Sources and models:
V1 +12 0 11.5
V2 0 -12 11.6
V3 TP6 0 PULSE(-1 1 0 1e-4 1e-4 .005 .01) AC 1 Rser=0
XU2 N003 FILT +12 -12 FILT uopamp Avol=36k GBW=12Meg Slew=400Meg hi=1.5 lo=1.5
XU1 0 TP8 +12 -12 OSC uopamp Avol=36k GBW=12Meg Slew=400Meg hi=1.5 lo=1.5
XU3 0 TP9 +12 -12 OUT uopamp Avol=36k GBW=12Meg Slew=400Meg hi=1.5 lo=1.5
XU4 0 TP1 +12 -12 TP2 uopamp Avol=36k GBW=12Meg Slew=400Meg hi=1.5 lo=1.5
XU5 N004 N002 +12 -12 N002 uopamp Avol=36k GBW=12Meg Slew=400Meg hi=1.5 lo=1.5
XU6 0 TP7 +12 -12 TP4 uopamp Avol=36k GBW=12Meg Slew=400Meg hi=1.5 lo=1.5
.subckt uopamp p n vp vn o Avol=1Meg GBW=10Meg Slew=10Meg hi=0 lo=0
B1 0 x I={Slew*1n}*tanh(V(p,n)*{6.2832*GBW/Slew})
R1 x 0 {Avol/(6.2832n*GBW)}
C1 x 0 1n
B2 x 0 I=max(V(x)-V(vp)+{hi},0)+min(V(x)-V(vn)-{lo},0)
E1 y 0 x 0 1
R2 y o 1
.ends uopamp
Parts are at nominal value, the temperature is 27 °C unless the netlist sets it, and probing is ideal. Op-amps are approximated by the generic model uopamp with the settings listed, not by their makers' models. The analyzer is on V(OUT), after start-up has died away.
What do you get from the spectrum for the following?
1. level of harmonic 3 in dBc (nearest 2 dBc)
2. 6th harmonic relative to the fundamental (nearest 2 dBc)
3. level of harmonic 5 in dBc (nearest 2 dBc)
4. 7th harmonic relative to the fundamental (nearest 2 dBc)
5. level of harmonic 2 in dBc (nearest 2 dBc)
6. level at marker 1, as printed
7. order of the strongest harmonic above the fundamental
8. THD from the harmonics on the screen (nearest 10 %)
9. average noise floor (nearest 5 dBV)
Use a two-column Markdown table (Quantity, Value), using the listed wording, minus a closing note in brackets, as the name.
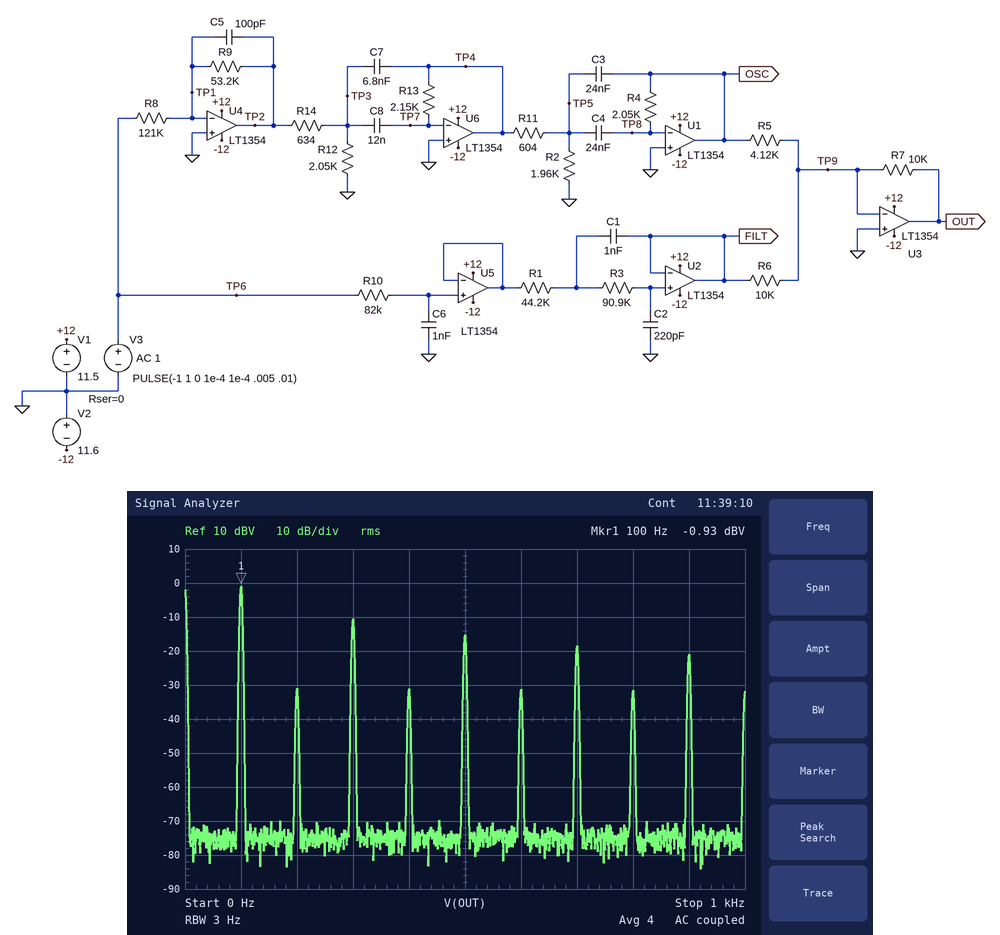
| Quantity | Value |
|---|---|
| level of harmonic 3 in dBc | -10 dBc |
| 6th harmonic relative to the fundamental | -30 dBc |
| level of harmonic 5 in dBc | -14 dBc |
| 7th harmonic relative to the fundamental | -18 dBc |
| level of harmonic 2 in dBc | -30 dBc |
| level at marker 1, as printed | -0.93 dBV |
| order of the strongest harmonic above the fundamental | 3 |
| THD from the harmonics on the screen | 40 % |
| average noise floor | -75 dBV |
